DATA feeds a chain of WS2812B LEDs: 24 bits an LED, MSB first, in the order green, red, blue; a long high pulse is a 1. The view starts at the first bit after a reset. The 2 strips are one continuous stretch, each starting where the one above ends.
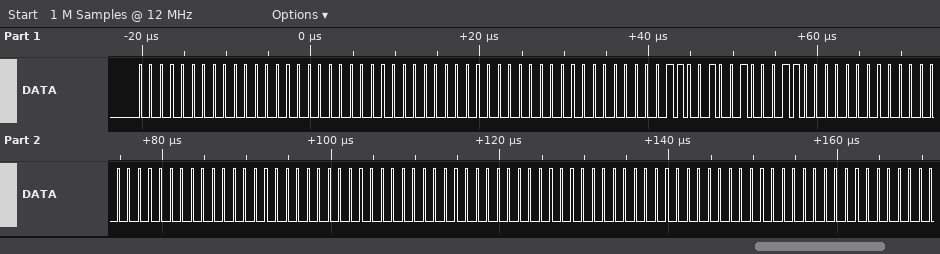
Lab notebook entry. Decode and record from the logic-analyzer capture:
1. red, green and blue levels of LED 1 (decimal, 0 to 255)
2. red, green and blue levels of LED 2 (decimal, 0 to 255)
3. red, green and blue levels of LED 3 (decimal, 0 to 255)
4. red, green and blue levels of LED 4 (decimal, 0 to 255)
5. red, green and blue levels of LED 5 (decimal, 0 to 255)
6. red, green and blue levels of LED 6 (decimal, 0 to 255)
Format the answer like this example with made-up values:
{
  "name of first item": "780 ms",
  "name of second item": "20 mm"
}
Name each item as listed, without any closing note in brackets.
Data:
{
  "red, green and blue levels of LED 1": "0, 0, 0",
  "red, green and blue levels of LED 2": "0, 0, 0",
  "red, green and blue levels of LED 3": "70, 50, 0",
  "red, green and blue levels of LED 4": "0, 0, 0",
  "red, green and blue levels of LED 5": "0, 0, 0",
  "red, green and blue levels of LED 6": "0, 0, 0"
}
